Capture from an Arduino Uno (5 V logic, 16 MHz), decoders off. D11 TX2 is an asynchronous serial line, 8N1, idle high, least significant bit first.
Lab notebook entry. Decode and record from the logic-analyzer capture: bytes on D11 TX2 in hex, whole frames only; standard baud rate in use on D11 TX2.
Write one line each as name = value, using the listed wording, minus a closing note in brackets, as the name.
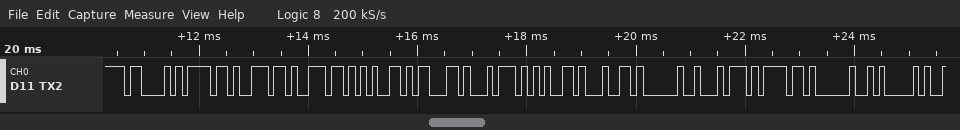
bytes on D11 TX2 in hex, whole frames only = 0x43 0x6F 0x6E 0x6E 0x65 0x63 0x74 0x65 0x64 0x20 0x74 0x6F 0x20 0x41
standard baud rate in use on D11 TX2 = 9600 baud
